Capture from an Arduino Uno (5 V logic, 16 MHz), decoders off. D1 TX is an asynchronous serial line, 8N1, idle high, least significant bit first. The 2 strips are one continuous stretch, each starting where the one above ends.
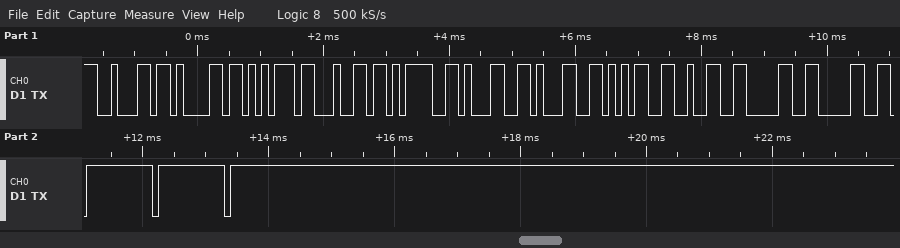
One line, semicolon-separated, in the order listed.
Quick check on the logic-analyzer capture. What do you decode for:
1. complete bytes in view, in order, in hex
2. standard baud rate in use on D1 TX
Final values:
0x62 0x61 0x75 0x64 0x3D 0x31 0x31 0x35 0x32 0x30 0x30 0xFF 0xFF 0xFF; 9600 baud
